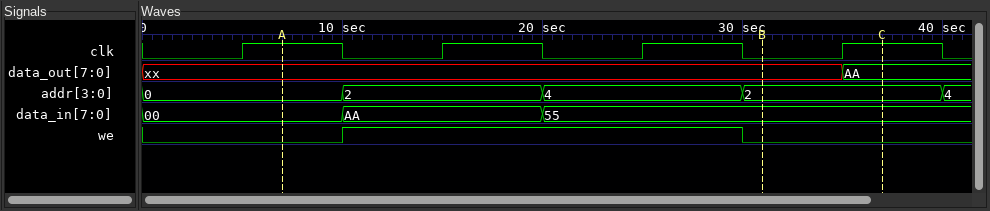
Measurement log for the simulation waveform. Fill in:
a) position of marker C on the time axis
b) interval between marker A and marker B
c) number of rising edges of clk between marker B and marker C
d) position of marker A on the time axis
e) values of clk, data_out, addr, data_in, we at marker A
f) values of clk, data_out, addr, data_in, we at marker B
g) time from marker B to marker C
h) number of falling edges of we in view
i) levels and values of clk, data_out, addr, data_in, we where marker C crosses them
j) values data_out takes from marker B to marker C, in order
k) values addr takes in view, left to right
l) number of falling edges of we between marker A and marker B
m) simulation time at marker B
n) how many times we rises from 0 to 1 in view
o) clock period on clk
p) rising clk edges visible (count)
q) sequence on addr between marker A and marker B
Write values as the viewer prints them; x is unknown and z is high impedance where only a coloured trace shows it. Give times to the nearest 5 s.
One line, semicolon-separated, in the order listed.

35 s; 25 s; 1; 5 s; clk=1, data_out=xx, addr=0, data_in=00, we=0; clk=0, data_out=xx, addr=2, data_in=55, we=0; 5 s; 1; clk=1, data_out=AA, addr=2, data_in=55, we=0; xx, AA; 0, 2, 4, 2, 4; 1; 30 s; 1; 10 s; 4; 0, 2, 4, 2
